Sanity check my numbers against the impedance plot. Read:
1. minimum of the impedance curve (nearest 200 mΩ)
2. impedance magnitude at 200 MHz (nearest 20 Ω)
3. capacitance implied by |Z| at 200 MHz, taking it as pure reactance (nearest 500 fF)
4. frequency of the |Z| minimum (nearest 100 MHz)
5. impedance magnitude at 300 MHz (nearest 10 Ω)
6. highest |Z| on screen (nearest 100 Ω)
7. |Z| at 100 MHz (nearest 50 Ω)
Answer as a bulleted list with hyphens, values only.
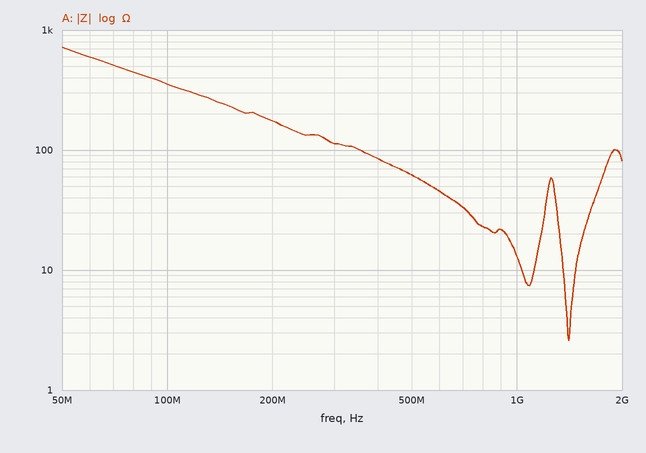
- 2.6 Ω
- 180 Ω
- 4.5 pF
- 1.4 GHz
- 110 Ω
- 700 Ω
- 350 Ω
